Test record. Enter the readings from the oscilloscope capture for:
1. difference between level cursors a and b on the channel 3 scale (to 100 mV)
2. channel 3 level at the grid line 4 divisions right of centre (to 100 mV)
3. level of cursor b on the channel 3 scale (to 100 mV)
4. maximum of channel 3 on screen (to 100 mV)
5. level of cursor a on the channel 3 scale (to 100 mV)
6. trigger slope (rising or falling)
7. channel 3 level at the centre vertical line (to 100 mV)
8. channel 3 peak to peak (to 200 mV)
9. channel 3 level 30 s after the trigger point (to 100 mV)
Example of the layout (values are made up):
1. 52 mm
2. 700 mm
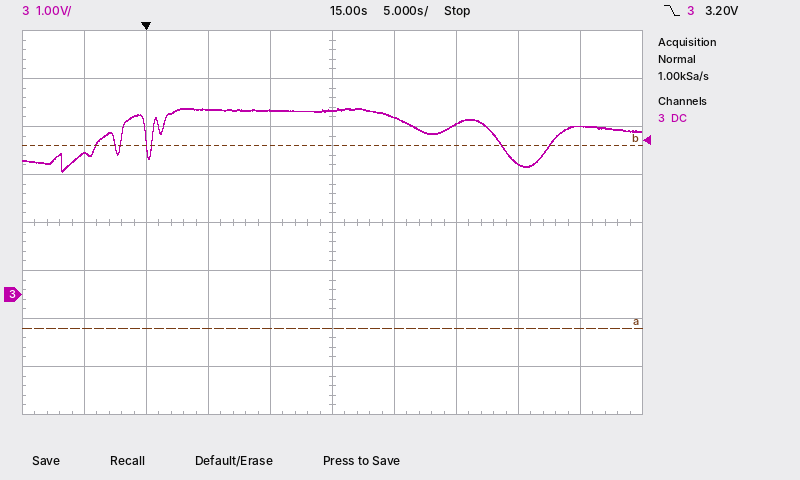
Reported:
1. 3.8 V
2. 3.5 V
3. 3.1 V
4. 3.9 V
5. -700 mV
6. falling
7. 3.8 V
8. 1.4 V
9. 2.7 V
